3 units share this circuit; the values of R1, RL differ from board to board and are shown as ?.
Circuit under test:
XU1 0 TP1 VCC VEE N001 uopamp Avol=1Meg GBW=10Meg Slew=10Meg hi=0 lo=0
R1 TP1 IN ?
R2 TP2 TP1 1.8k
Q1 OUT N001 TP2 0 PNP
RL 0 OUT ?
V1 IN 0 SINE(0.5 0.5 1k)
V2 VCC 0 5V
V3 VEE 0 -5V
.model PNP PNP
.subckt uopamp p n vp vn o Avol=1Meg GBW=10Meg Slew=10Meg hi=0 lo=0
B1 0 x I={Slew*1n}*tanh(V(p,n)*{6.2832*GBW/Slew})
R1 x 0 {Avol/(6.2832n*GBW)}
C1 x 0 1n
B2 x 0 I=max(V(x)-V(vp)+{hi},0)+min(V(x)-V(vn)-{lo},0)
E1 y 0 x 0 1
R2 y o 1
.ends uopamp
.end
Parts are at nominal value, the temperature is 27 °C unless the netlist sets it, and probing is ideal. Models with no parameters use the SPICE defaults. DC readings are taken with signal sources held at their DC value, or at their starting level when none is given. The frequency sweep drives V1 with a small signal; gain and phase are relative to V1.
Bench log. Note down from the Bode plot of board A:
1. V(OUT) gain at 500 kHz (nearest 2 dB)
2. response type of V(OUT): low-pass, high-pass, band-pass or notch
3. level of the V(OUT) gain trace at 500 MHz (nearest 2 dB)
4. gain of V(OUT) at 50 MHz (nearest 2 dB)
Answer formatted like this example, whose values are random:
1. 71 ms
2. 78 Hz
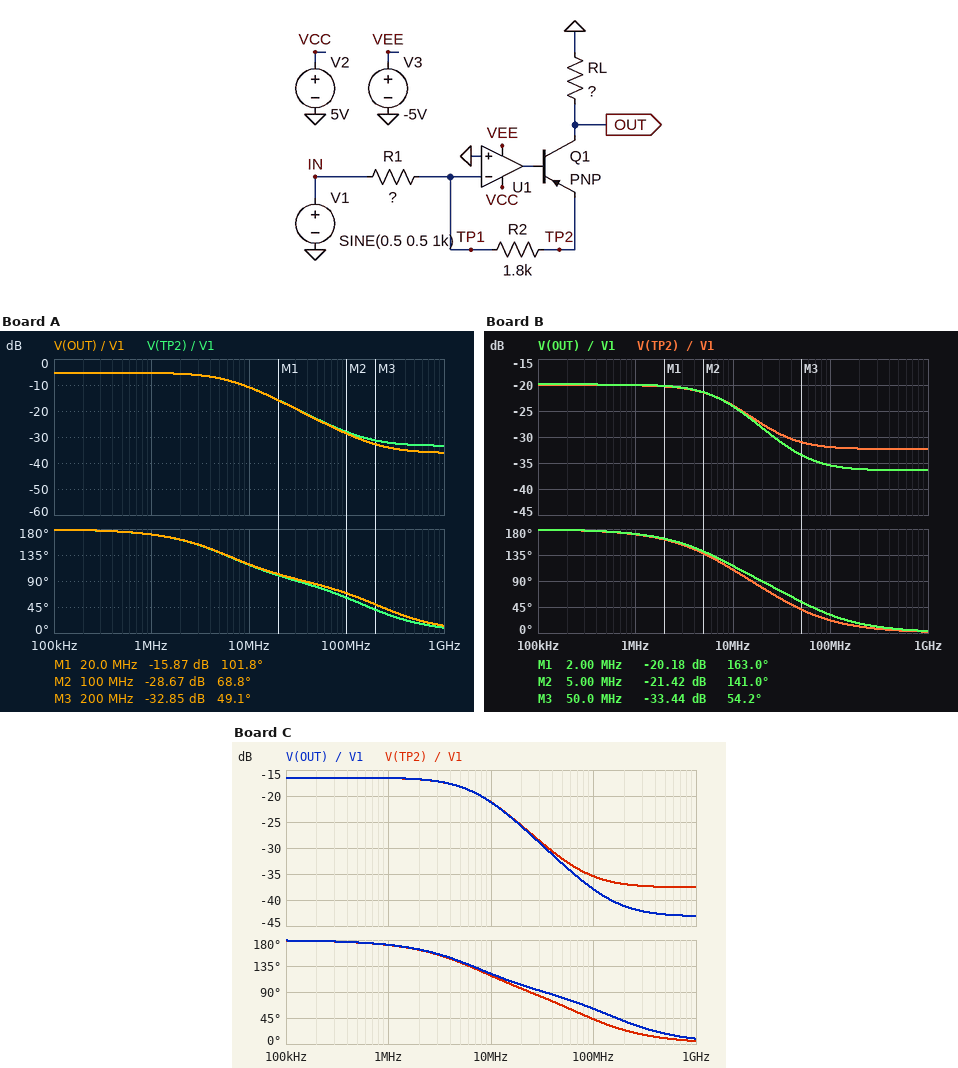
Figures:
1. -6 dB
2. low-pass
3. -36 dB
4. -24 dB
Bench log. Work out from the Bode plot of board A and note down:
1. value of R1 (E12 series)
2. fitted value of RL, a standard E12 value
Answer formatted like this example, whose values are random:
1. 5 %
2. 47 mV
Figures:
1. 3.3 kΩ
2. 1.8 kΩ
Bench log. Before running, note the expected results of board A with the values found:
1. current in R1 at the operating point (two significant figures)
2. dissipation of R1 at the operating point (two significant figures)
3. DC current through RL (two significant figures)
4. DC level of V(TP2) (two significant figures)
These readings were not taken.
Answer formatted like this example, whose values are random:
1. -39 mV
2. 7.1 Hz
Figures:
1. 150 µA
2. 76 µW
3. 160 µA
4. -270 mV
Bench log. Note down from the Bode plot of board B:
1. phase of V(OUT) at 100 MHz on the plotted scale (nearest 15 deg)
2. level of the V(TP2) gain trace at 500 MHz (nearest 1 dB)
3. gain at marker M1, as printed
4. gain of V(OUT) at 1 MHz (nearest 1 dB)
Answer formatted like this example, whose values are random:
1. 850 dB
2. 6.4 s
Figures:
1. 30 deg
2. -32 dB
3. -20.18 dB
4. -20 dB
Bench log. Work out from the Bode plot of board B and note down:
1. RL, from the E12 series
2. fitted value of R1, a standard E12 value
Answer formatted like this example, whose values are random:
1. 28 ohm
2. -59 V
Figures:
1. 1.5 kΩ
2. 18 kΩ
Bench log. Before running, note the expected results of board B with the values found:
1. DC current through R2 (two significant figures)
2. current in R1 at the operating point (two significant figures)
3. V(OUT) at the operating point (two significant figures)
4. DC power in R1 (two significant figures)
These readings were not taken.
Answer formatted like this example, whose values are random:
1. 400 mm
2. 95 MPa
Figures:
1. 28 µA
2. 28 µA
3. -59 mV
4. 14 µW
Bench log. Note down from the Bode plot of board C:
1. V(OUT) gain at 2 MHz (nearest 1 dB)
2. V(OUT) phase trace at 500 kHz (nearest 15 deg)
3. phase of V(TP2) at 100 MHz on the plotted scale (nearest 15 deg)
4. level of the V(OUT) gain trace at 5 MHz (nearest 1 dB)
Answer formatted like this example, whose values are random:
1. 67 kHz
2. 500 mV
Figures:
1. -17 dB
2. 180 deg
3. 45 deg
4. -18 dB
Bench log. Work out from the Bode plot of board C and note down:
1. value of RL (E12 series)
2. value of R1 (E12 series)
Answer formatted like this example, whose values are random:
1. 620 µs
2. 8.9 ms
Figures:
1. 470 Ω
2. 12 kΩ
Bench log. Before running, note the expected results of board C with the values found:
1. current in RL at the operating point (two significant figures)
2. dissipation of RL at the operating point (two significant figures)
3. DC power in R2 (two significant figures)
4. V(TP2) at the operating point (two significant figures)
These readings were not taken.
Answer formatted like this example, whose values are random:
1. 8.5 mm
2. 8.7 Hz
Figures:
1. 170 µA
2. 13 µW
3. 3.1 µW
4. -75 mV
